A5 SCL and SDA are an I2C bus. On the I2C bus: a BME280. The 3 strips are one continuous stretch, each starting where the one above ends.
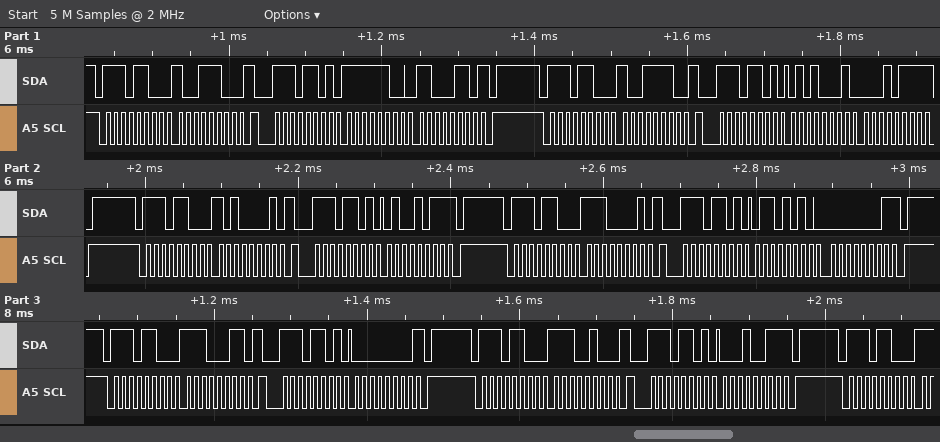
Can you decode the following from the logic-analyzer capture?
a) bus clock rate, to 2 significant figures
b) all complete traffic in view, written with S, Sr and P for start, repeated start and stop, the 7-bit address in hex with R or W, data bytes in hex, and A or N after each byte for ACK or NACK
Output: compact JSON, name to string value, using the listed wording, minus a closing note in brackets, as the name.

{"bus clock rate, to 2 significant figures": "100 kHz", "all complete traffic in view, written with S, Sr and P for start, repeated start and stop, the 7-bit address in hex with R or W, data bytes in hex, and A or N after each byte for ACK or NACK": "S 76W A 9C A Sr 76R A FC A C6 N P S 76W A 9E A Sr 76R A 51 A 17 N P S 76W A A1 A Sr 76R A 4B N P S 76W A E1 A Sr 76R A 6A A 01 N P S 76W A E3 A Sr 76R A 00 N P S 76W A E4 A Sr 76R A 13 N P S 76W A"}
